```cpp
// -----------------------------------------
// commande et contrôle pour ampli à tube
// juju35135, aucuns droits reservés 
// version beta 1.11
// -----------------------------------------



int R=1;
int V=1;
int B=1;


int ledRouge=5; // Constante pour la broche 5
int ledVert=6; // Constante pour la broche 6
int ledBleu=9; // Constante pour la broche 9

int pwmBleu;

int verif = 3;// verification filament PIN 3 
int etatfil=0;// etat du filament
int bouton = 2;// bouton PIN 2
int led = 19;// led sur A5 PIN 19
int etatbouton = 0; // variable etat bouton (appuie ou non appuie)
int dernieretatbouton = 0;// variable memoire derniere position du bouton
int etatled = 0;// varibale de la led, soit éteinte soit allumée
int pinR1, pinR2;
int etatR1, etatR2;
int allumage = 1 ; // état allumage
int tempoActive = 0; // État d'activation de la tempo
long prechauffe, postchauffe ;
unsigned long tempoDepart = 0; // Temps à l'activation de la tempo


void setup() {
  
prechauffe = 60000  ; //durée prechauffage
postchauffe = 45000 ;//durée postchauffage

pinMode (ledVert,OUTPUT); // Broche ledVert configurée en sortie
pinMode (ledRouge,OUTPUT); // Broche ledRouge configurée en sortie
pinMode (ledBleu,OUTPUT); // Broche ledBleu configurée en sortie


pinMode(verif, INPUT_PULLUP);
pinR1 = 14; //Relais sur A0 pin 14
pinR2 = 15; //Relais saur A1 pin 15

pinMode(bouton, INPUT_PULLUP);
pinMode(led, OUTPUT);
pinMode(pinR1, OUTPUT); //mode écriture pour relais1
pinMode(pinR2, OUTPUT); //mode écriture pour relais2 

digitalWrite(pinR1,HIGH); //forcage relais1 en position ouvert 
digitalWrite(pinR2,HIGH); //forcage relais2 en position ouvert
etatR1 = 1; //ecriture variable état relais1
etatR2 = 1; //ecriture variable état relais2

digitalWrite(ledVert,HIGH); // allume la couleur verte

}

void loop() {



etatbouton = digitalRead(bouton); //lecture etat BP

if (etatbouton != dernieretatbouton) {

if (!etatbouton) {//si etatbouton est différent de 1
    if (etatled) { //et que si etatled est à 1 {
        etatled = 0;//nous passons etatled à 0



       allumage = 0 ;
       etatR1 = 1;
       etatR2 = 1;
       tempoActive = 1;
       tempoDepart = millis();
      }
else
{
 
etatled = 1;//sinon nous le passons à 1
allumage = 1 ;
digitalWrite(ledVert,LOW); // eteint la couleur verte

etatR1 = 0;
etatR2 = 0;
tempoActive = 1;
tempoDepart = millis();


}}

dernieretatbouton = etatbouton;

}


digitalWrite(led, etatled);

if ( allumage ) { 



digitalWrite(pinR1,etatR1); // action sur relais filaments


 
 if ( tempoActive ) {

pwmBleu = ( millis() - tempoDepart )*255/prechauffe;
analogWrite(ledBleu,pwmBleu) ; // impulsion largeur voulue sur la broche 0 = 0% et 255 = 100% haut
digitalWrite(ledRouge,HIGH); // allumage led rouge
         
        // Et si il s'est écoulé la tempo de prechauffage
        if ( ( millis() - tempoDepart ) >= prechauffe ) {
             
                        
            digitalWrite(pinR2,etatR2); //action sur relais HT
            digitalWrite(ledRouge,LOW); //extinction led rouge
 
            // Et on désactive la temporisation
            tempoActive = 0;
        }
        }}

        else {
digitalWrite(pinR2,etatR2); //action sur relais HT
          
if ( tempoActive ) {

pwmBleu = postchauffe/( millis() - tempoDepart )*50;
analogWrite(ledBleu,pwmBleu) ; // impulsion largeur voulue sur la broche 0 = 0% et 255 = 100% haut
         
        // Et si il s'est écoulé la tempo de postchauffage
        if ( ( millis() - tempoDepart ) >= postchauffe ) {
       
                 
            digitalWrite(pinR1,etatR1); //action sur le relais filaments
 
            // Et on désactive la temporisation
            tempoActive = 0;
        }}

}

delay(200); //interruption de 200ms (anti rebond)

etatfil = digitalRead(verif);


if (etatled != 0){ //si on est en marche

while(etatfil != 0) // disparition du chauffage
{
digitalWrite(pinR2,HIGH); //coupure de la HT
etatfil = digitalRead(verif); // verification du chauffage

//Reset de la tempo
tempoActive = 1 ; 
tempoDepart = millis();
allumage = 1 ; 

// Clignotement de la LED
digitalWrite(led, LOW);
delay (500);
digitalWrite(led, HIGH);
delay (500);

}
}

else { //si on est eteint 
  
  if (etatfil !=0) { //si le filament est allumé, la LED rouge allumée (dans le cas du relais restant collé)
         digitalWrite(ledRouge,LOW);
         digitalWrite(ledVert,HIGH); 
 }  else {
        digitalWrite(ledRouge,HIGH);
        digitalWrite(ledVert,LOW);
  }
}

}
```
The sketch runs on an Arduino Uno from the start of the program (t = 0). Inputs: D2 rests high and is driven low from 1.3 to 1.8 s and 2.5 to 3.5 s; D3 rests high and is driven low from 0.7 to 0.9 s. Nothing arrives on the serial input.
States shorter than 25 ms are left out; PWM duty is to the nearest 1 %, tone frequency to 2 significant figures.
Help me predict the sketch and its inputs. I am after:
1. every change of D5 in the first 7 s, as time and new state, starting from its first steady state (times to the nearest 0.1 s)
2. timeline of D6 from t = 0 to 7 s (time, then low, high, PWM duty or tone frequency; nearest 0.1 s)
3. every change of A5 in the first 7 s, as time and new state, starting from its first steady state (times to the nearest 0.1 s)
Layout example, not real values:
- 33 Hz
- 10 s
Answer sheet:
- 0 s low; 0.8 s high; 1 s low; 1.4 s high
- 0 s high; 0.8 s low; 1 s high; 1.4 s low
- 0 s low; 1.4 s high; 1.6 s low; 2.1 s high; 2.6 s low; 3.1 s high; 3.6 s low; 4.1 s high; 4.6 s low; 5.1 s high; 5.6 s low; 6.1 s high; 6.6 s low
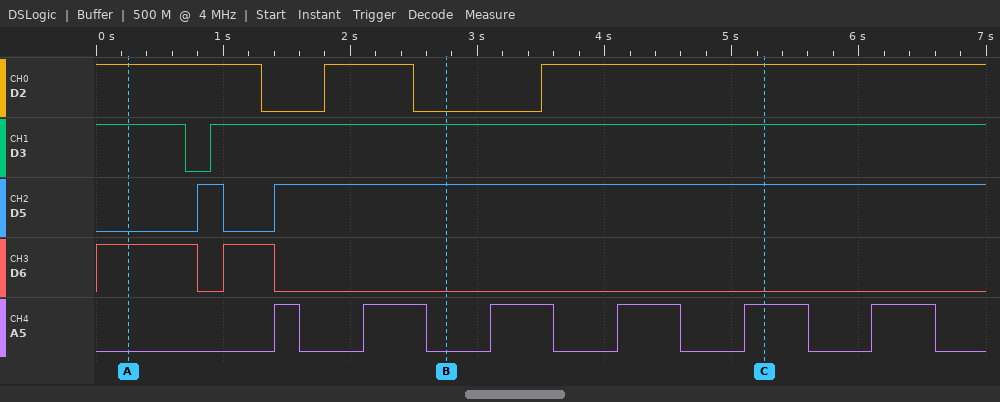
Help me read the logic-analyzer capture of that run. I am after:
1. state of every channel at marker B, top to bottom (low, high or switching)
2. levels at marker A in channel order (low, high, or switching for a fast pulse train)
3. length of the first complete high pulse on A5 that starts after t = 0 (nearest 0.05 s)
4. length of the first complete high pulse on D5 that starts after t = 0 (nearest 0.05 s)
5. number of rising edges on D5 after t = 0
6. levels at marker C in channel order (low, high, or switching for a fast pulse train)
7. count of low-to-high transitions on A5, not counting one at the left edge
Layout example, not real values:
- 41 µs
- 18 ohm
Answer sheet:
- D2 low, D3 high, D5 high, D6 low, A5 low
- D2 high, D3 high, D5 low, D6 high, A5 low
- 0.20 s
- 0.20 s
- 2
- D2 high, D3 high, D5 high, D6 low, A5 high
- 6
